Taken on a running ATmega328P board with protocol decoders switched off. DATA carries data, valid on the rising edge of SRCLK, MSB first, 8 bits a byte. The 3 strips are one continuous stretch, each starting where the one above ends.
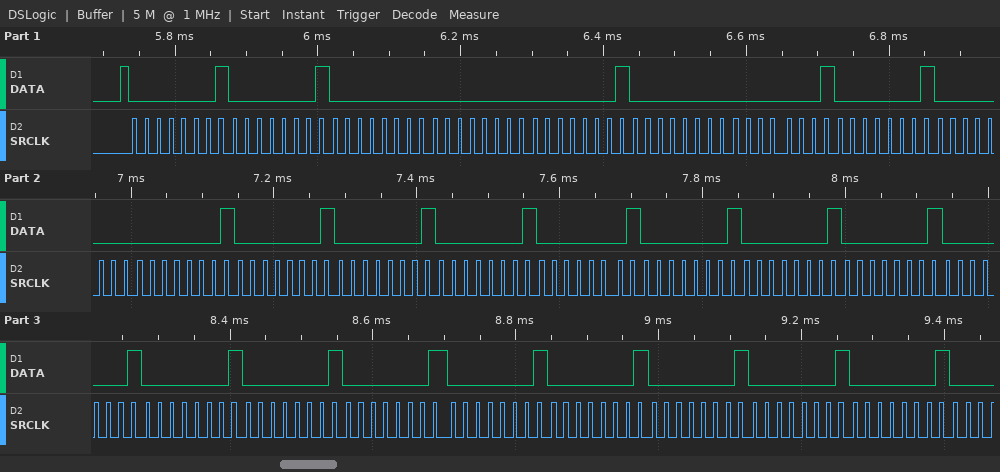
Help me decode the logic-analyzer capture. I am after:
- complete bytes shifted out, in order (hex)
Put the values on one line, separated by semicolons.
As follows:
01 01 00 00 01 00 01 01 00 01 01 01 01 01 01 01 01 01 01 01 01 01 01 01 01 01
